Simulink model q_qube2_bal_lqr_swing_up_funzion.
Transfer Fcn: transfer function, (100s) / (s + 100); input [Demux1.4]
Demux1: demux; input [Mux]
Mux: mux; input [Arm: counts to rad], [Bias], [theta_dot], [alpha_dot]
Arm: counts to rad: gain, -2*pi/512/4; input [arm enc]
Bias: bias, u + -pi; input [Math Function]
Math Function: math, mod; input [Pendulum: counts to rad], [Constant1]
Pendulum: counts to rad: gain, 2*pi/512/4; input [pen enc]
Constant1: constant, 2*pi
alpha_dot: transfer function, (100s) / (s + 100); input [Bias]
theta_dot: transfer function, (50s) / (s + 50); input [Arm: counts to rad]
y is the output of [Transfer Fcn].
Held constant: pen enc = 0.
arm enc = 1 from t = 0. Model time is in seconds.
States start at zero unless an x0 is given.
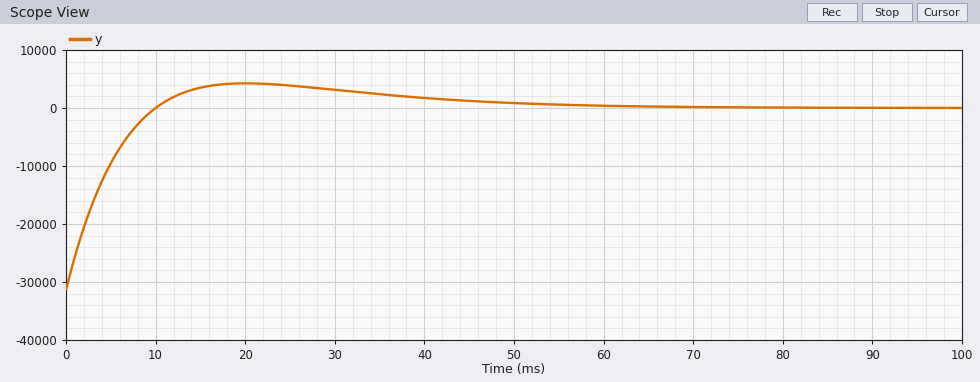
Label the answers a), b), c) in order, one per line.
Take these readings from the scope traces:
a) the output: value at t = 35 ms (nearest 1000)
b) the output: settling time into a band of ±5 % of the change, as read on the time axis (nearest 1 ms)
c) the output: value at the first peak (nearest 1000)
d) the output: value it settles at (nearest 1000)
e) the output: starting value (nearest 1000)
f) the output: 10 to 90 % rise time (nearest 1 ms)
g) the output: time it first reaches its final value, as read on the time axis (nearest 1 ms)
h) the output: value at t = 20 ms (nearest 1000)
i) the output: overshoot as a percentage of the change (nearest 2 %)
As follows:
a) 2000
b) 41 ms
c) 4000
d) 0
e) -31000
f) 7 ms
g) 10 ms
h) 4000
i) 14 %
